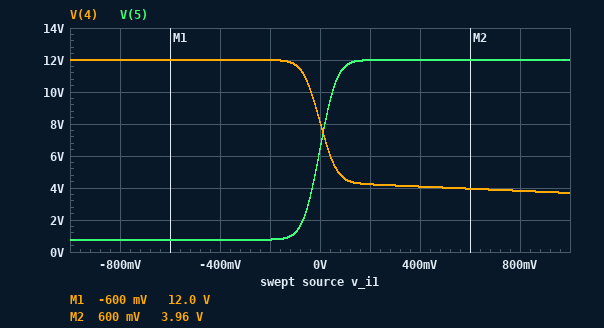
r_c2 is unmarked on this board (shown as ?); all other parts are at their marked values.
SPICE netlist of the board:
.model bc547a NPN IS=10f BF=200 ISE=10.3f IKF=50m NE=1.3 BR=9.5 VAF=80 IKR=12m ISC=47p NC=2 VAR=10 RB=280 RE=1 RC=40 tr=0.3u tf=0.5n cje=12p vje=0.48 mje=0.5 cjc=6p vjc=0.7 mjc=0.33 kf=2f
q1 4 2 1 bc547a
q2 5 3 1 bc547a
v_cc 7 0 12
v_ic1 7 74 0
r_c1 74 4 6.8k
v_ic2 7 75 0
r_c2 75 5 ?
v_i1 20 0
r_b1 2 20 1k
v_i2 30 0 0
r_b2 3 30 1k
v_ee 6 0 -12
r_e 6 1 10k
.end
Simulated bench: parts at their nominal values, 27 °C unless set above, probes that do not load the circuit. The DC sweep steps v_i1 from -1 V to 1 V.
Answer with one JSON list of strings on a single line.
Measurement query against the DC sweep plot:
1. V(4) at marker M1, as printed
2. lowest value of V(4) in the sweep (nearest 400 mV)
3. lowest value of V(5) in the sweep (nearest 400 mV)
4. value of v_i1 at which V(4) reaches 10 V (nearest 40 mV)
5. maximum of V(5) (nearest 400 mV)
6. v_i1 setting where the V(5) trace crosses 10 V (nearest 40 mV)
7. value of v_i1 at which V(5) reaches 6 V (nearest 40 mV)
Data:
["12.0 V", "3.6 V", "800 mV", "-40 mV", "12.0 V", "40 mV", "0 V"]
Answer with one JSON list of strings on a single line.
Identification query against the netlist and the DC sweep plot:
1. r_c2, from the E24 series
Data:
["10 kΩ"]
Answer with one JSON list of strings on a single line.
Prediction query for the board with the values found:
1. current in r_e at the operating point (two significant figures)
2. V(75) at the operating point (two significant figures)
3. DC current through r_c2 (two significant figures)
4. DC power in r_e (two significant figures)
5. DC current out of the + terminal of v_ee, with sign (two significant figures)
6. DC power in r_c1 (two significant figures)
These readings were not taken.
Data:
["1.1 mA", "12 V", "560 µA", "13 mW", "-1.1 mA", "2.2 mW"]
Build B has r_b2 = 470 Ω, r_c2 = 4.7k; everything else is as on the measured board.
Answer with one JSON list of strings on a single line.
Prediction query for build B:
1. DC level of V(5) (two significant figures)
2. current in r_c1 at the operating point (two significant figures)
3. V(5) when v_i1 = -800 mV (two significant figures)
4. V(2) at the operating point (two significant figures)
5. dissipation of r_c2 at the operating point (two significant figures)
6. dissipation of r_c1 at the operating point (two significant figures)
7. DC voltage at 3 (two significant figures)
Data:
["9.2 V", "540 µA", "6.7 V", "-4.4 mV", "1.6 mW", "2.0 mW", "-2.2 mV"]
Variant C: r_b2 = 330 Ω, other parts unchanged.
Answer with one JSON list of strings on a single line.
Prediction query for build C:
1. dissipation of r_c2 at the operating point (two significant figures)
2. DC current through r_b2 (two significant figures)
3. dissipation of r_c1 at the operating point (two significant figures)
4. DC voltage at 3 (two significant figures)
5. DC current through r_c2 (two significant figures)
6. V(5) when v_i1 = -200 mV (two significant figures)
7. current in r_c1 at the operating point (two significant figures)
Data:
["3.4 mW", "4.9 µA", "2.0 mW", "-1.6 mV", "580 µA", "770 mV", "540 µA"]
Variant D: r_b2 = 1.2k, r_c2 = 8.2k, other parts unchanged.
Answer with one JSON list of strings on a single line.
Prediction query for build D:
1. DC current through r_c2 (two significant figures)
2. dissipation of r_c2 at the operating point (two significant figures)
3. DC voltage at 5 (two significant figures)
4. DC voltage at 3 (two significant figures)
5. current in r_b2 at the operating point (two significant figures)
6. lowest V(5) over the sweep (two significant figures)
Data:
["550 µA", "2.5 mW", "7.5 V", "-5.5 mV", "4.6 µA", "2.8 V"]
